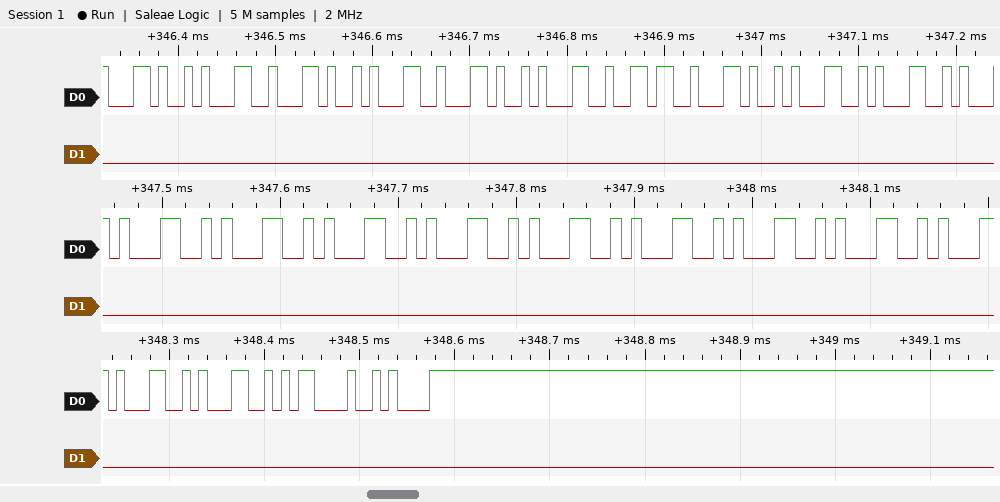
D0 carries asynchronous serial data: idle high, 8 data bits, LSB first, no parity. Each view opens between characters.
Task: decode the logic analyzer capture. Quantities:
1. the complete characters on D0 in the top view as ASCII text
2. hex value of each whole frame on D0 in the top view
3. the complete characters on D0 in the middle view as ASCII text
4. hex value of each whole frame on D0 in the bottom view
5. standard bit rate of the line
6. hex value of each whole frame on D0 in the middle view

",1,1,16,11"
2C, 31, 2C, 31, 2C, 31, 36, 2C, 31, 31
"11111111"
31, 31, 0D, 0A
115200 baud
31, 31, 31, 31, 31, 31, 31, 31
